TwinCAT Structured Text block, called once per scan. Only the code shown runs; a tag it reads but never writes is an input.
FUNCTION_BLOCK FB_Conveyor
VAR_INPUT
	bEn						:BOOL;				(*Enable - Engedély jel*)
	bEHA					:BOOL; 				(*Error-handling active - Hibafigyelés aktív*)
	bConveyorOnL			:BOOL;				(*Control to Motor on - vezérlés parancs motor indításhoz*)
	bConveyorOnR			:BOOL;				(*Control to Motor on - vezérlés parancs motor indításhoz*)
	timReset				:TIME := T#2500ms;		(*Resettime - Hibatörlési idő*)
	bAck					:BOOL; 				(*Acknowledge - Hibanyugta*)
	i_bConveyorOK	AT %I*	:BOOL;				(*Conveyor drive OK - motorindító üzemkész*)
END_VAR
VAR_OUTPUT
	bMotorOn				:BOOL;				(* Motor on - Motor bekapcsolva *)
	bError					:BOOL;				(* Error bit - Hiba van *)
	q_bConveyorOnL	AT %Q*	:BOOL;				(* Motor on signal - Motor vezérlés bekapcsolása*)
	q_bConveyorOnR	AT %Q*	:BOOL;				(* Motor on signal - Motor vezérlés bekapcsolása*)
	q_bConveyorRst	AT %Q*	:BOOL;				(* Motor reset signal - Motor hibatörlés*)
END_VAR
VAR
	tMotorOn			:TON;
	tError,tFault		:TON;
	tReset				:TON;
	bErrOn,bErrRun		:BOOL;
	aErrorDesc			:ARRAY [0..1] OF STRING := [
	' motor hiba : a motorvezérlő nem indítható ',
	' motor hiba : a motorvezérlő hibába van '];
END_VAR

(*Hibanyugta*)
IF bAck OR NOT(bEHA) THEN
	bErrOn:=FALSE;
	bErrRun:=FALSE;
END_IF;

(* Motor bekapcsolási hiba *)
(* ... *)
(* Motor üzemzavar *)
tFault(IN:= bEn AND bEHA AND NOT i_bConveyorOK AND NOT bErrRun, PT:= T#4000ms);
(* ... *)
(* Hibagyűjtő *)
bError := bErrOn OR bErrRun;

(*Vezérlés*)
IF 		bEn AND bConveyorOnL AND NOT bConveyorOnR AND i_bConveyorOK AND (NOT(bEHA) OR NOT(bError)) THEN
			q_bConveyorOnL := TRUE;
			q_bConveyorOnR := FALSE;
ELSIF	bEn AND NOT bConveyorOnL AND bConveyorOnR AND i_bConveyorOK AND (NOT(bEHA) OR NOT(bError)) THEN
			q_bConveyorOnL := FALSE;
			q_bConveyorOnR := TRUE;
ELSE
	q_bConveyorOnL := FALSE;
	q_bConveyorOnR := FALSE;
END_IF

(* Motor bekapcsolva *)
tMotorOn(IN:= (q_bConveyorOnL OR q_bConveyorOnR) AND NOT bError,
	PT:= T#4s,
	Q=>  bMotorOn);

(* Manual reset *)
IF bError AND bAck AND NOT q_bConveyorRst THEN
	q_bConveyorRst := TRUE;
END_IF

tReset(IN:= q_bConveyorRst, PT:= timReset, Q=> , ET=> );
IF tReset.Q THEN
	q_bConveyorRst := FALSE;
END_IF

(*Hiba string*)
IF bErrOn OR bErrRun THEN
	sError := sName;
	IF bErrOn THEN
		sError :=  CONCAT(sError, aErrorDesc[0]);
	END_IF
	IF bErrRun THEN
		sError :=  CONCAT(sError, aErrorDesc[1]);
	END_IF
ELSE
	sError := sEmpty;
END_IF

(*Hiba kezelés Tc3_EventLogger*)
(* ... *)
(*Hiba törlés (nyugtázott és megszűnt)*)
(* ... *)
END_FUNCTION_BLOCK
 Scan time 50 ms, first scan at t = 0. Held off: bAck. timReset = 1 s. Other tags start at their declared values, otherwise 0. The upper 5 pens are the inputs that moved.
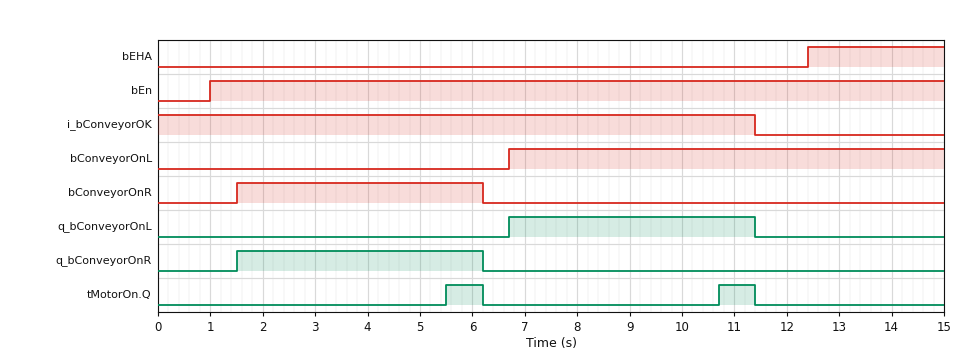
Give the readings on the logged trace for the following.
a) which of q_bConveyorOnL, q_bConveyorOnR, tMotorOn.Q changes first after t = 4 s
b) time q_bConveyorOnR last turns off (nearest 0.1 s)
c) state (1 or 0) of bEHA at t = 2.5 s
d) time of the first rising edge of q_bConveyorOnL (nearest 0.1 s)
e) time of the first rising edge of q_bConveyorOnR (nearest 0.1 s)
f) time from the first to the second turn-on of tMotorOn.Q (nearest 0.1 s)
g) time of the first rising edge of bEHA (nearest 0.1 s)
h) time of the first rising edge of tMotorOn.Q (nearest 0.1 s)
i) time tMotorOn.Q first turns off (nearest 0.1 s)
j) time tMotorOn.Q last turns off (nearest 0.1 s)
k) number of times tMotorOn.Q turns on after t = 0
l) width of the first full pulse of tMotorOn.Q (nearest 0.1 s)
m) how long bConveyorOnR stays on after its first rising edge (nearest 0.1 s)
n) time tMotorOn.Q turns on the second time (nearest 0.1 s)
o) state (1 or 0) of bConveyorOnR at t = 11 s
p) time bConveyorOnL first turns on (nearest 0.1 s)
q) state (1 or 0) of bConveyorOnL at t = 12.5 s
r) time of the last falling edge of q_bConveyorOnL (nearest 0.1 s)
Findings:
tMotorOn.Q
6.2 s
0
6.7 s
1.5 s
5.2 s
12.4 s
5.5 s
6.2 s
11.4 s
2
0.7 s
4.7 s
10.7 s
0
6.7 s
1
11.4 s
